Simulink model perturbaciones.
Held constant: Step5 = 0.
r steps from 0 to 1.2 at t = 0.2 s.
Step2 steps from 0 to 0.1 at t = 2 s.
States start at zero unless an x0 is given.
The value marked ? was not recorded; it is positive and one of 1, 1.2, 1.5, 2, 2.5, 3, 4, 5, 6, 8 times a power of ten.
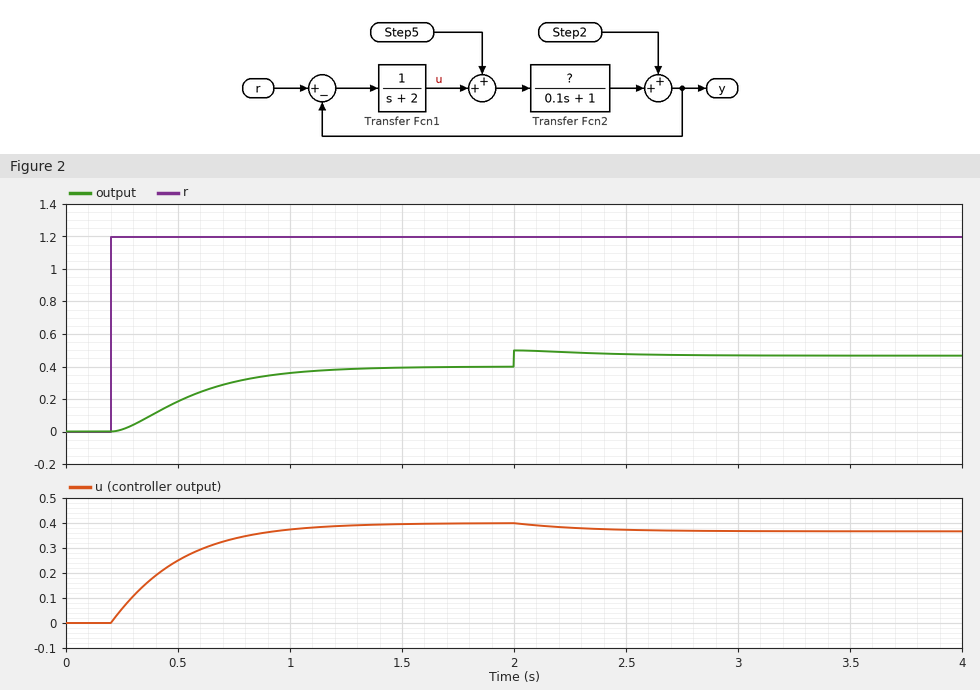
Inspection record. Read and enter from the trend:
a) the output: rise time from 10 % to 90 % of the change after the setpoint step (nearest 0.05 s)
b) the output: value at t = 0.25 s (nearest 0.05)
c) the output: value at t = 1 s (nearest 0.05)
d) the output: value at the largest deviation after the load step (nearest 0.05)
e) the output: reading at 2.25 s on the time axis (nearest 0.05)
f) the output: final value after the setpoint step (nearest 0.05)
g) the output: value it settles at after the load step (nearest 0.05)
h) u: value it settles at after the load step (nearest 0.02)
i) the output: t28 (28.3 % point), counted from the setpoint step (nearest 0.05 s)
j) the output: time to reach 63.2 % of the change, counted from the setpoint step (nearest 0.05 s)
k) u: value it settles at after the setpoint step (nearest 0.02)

0.70 s
0.00
0.35
0.50
0.50
0.40
0.45
0.36
0.20 s
0.40 s
0.40
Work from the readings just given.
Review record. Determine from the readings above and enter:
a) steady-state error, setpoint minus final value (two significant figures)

0.80
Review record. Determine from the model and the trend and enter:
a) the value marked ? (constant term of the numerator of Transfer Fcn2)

1
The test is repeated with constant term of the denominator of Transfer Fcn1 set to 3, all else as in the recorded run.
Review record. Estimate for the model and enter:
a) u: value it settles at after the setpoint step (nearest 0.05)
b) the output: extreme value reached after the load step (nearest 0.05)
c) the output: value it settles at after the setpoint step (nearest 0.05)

0.30
0.40
0.30
